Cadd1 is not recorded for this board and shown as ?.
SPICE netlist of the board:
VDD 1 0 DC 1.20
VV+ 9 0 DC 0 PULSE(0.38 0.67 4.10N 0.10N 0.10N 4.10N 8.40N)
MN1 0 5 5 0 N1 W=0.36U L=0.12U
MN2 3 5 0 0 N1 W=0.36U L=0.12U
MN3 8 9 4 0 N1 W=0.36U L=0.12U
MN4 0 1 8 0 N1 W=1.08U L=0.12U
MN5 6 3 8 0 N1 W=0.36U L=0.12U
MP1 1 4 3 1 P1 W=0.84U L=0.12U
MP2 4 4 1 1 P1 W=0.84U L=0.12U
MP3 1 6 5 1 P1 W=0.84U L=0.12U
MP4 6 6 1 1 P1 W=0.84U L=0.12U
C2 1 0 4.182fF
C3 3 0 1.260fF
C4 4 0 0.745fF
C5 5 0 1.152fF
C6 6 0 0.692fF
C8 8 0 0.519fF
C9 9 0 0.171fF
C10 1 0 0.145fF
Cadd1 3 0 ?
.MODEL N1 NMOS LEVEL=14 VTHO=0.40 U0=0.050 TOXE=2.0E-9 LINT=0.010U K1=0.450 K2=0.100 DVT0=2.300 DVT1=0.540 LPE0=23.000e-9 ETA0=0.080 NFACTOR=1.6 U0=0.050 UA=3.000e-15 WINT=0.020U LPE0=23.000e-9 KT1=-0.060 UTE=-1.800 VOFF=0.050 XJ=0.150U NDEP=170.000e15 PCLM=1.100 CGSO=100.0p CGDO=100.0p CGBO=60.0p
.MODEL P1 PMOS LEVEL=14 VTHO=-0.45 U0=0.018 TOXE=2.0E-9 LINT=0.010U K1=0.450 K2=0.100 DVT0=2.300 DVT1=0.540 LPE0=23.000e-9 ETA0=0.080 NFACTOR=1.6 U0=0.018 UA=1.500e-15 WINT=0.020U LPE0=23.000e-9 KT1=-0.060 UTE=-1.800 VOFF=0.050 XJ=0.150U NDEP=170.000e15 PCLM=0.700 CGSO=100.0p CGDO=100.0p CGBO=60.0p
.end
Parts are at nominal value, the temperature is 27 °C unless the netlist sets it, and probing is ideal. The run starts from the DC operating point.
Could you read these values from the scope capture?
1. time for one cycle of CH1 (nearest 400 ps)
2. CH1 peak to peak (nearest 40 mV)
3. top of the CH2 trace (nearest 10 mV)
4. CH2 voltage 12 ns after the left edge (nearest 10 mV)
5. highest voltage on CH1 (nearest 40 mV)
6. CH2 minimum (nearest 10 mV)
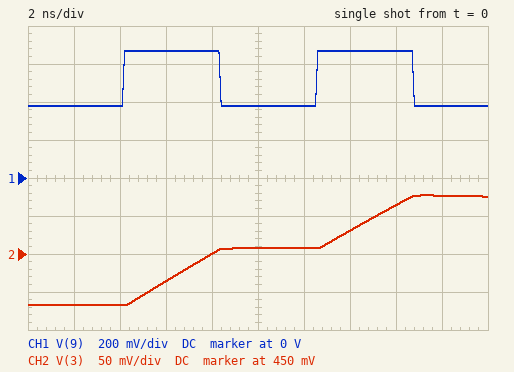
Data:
8.4 ns
280 mV
530 mV
460 mV
680 mV
380 mV
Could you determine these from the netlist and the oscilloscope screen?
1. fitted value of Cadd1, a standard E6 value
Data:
470 fF
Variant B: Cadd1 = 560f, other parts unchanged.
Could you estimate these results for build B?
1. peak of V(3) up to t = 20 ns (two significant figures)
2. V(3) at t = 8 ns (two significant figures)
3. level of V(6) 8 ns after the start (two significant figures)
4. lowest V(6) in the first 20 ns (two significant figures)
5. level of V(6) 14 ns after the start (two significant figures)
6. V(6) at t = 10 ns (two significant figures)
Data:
510 mV
440 mV
740 mV
640 mV
700 mV
720 mV
